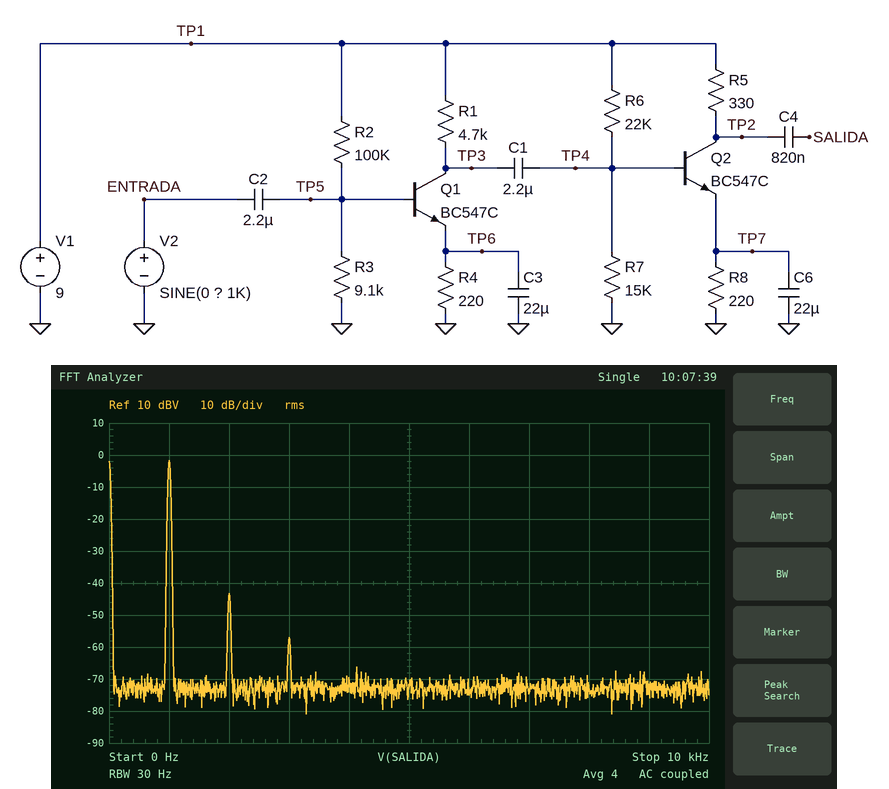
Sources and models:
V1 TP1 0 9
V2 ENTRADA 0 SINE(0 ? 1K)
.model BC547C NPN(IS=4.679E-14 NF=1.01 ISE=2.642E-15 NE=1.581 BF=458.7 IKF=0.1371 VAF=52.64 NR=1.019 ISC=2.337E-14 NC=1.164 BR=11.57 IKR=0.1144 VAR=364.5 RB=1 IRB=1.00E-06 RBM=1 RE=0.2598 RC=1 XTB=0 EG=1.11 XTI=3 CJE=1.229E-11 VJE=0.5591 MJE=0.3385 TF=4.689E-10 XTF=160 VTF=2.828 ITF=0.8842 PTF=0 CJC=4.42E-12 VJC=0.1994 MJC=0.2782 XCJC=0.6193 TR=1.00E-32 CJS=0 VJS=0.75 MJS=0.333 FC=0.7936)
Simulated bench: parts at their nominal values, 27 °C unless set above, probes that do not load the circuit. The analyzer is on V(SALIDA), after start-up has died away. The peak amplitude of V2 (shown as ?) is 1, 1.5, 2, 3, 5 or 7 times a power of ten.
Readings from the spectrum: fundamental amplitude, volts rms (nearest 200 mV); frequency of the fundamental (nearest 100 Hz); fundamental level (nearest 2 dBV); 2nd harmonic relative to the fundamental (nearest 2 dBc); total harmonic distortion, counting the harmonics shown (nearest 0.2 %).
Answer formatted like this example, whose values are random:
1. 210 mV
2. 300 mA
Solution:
1. 800 mV
2. 1.0 kHz
3. -2 dBV
4. -42 dBc
5. 0.8 %
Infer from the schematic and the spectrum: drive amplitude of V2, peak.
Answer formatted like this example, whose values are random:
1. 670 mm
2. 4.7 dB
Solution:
1. 700 µV
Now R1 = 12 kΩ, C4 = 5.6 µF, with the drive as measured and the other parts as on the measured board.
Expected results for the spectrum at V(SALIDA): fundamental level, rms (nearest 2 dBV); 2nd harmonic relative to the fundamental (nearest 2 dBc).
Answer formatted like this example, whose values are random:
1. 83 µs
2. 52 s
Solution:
1. 0 dBV
2. -36 dBc
